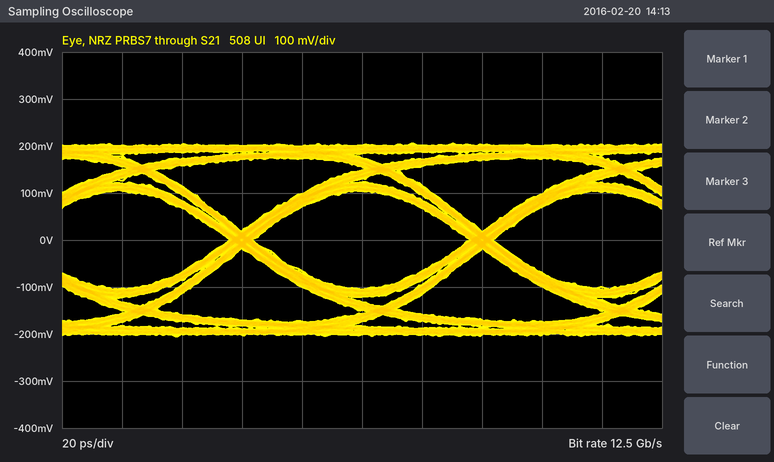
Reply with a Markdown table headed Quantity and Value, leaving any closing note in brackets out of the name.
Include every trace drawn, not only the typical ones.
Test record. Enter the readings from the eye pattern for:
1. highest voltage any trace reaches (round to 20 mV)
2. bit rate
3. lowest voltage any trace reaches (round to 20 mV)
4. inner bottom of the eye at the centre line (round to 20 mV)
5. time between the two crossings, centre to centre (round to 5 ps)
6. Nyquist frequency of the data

| Quantity | Value |
|---|---|
| highest voltage any trace reaches | 200 mV |
| bit rate | 12.5 Gb/s |
| lowest voltage any trace reaches | -200 mV |
| inner bottom of the eye at the centre line | -100 mV |
| time between the two crossings, centre to centre | 80 ps |
| Nyquist frequency of the data | 6.25 GHz |
